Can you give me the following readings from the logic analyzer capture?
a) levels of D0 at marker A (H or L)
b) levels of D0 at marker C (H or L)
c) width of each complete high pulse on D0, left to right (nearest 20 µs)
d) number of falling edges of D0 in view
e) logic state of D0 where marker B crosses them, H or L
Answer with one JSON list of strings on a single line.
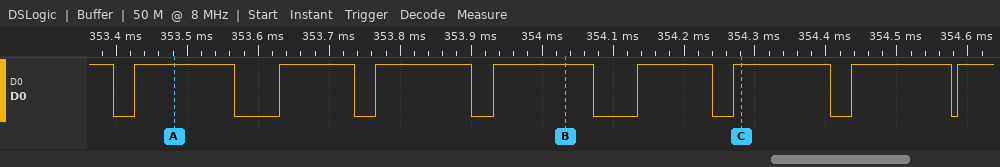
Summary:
["D0=H", "D0=H", "140 µs, 100 µs, 140 µs, 140 µs, 100 µs, 140 µs, 140 µs", "8", "D0=H"]
